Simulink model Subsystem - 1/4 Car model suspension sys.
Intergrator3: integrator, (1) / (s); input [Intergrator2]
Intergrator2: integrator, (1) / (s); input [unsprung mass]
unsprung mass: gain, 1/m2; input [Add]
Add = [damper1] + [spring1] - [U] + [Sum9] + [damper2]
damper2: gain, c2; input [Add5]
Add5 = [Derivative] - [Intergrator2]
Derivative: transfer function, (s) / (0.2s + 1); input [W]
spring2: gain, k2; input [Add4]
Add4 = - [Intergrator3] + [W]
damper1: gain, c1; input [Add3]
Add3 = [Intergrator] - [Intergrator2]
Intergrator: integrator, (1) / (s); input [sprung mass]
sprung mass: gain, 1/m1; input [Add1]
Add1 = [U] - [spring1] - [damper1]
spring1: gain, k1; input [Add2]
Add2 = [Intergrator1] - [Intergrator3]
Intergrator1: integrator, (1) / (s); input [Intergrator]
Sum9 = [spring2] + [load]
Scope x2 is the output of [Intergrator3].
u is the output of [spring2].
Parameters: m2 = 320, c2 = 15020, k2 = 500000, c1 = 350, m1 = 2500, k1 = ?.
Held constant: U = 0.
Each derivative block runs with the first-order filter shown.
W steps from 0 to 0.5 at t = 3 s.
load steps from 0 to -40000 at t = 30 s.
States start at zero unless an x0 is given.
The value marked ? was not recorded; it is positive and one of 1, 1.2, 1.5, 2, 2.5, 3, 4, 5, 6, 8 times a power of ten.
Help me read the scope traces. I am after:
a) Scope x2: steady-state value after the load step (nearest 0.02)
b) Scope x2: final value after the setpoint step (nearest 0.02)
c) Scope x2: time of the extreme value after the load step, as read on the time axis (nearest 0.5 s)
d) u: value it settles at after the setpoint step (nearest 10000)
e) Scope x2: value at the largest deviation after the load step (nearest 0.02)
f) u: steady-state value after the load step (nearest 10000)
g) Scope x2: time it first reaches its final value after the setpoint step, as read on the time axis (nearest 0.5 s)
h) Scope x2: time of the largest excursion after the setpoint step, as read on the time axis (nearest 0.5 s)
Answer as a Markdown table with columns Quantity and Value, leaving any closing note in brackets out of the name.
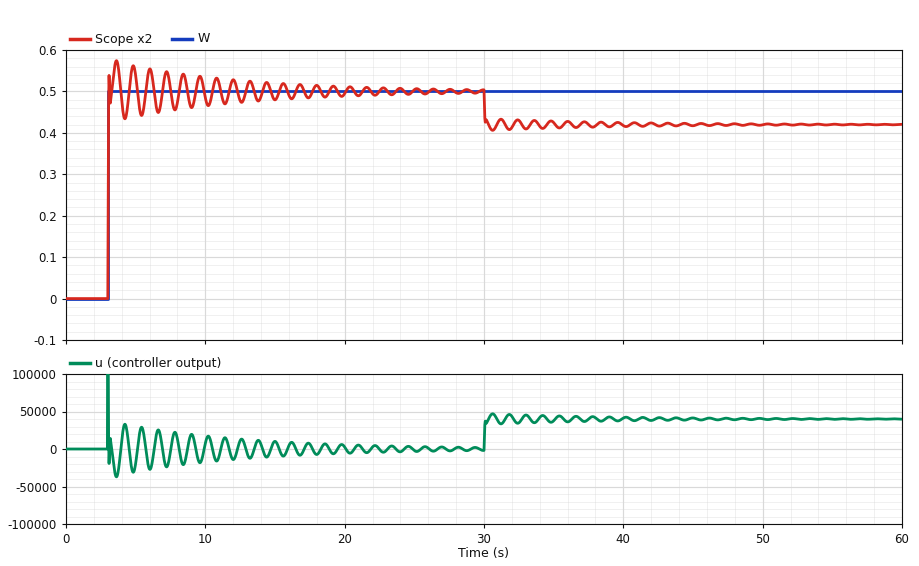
| Quantity | Value |
|---|---|
| Scope x2: steady-state value after the load step | 0.42 |
| Scope x2: final value after the setpoint step | 0.50 |
| Scope x2: time of the extreme value after the load step, as read on the time axis | 30.5 s |
| u: value it settles at after the setpoint step | 0 |
| Scope x2: value at the largest deviation after the load step | 0.40 |
| u: steady-state value after the load step | 40000 |
| Scope x2: time it first reaches its final value after the setpoint step, as read on the time axis | 3.0 s |
| Scope x2: time of the largest excursion after the setpoint step, as read on the time axis | 3.5 s |
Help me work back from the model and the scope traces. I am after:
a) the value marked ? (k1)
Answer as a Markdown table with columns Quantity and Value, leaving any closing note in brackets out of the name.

| Quantity | Value |
|---|---|
| the value marked ? | 80000 |
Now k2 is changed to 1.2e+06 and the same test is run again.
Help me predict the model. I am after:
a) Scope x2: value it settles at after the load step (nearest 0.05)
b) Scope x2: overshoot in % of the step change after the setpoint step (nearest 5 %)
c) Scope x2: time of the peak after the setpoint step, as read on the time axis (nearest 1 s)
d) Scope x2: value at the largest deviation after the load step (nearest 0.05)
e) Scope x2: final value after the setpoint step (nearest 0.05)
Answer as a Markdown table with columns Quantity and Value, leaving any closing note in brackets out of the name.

| Quantity | Value |
|---|---|
| Scope x2: value it settles at after the load step | 0.45 |
| Scope x2: overshoot in % of the step change after the setpoint step | 25 % |
| Scope x2: time of the peak after the setpoint step, as read on the time axis | 3 s |
| Scope x2: value at the largest deviation after the load step | 0.45 |
| Scope x2: final value after the setpoint step | 0.50 |
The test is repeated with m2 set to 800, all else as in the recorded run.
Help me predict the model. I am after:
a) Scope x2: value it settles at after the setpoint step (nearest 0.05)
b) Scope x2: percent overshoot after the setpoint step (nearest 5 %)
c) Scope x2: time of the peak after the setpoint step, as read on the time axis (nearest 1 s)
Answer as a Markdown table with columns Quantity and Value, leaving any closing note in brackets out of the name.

| Quantity | Value |
|---|---|
| Scope x2: value it settles at after the setpoint step | 0.50 |
| Scope x2: percent overshoot after the setpoint step | 25 % |
| Scope x2: time of the peak after the setpoint step, as read on the time axis | 3 s |
